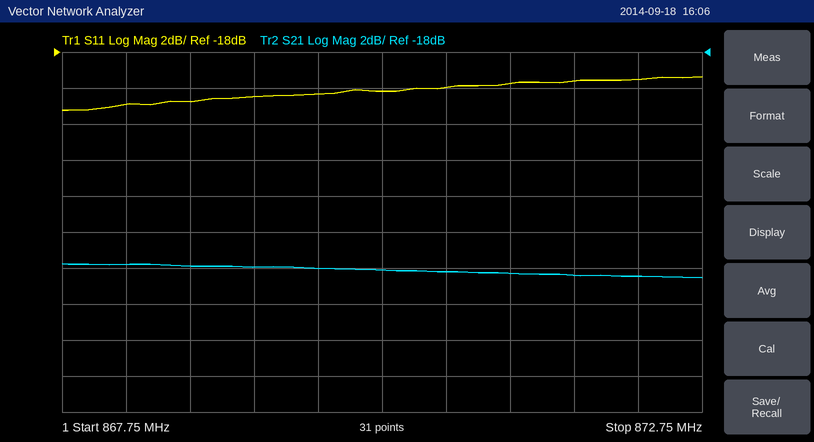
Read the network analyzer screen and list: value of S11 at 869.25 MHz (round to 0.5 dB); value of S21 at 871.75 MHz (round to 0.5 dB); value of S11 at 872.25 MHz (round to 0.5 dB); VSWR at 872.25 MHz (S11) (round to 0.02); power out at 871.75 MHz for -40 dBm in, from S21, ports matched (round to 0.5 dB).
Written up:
-20.5 dB
-30.5 dB
-19.5 dB
1.24
-70.5 dBm
